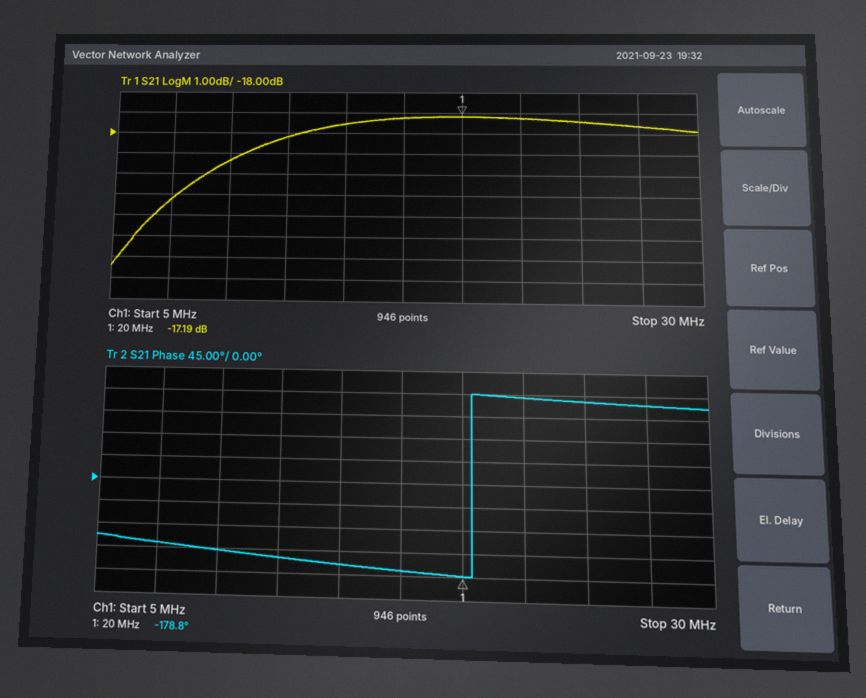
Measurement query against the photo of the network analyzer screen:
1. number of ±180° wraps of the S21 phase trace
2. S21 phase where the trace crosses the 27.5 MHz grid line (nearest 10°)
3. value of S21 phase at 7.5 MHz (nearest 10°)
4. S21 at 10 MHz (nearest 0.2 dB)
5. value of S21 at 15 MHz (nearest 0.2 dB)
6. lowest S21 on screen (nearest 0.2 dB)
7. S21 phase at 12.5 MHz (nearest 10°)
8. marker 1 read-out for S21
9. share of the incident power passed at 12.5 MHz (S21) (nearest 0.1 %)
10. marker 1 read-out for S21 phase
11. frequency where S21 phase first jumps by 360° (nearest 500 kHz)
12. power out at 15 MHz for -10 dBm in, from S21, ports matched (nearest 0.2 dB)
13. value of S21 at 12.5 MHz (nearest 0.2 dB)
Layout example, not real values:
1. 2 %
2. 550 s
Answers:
1. 1
2. 160°
3. -130°
4. -19.4 dB
5. -17.6 dB
6. -24.4 dB
7. -150°
8. -17.19 dB
9. 1.5 %
10. -178.8°
11. 20.5 MHz
12. -27.6 dBm
13. -18.2 dB
